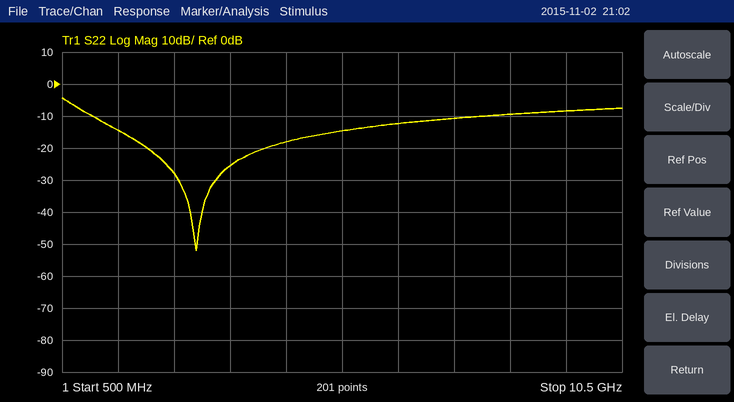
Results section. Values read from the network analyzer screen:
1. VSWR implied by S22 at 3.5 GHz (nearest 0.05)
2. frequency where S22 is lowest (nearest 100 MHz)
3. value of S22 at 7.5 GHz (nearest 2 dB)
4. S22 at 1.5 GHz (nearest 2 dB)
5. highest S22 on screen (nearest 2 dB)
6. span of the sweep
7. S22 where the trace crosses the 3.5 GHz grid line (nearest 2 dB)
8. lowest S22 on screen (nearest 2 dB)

1.10
2.9 GHz
-10 dB
-14 dB
-4 dB
10 GHz
-26 dB
-52 dB
